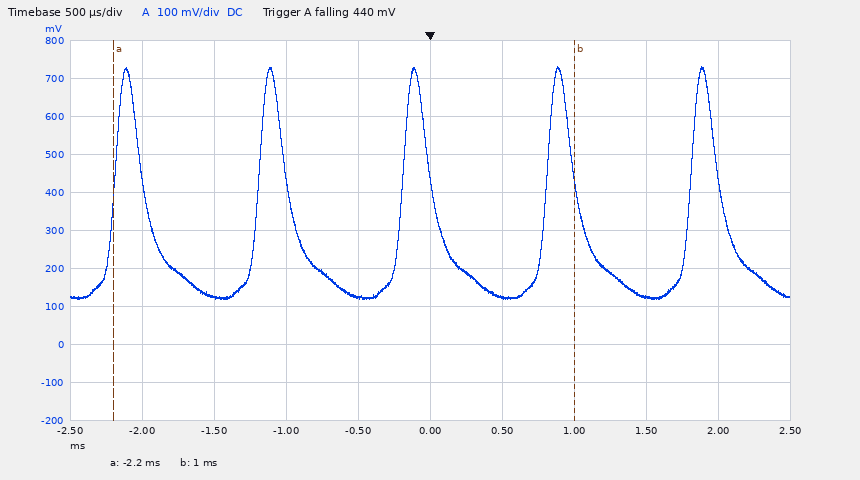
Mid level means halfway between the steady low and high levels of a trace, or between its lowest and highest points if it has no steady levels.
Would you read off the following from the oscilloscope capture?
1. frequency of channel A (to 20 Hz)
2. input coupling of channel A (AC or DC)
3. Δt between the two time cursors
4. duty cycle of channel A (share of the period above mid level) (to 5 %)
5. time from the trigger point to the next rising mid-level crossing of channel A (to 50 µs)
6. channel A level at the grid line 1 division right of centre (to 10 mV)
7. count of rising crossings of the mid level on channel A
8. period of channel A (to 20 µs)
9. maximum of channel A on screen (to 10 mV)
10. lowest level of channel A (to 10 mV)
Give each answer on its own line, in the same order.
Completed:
1.00 kHz
DC
3.20 ms
20 %
800 µs
120 mV
5
1.00 ms
730 mV
120 mV
